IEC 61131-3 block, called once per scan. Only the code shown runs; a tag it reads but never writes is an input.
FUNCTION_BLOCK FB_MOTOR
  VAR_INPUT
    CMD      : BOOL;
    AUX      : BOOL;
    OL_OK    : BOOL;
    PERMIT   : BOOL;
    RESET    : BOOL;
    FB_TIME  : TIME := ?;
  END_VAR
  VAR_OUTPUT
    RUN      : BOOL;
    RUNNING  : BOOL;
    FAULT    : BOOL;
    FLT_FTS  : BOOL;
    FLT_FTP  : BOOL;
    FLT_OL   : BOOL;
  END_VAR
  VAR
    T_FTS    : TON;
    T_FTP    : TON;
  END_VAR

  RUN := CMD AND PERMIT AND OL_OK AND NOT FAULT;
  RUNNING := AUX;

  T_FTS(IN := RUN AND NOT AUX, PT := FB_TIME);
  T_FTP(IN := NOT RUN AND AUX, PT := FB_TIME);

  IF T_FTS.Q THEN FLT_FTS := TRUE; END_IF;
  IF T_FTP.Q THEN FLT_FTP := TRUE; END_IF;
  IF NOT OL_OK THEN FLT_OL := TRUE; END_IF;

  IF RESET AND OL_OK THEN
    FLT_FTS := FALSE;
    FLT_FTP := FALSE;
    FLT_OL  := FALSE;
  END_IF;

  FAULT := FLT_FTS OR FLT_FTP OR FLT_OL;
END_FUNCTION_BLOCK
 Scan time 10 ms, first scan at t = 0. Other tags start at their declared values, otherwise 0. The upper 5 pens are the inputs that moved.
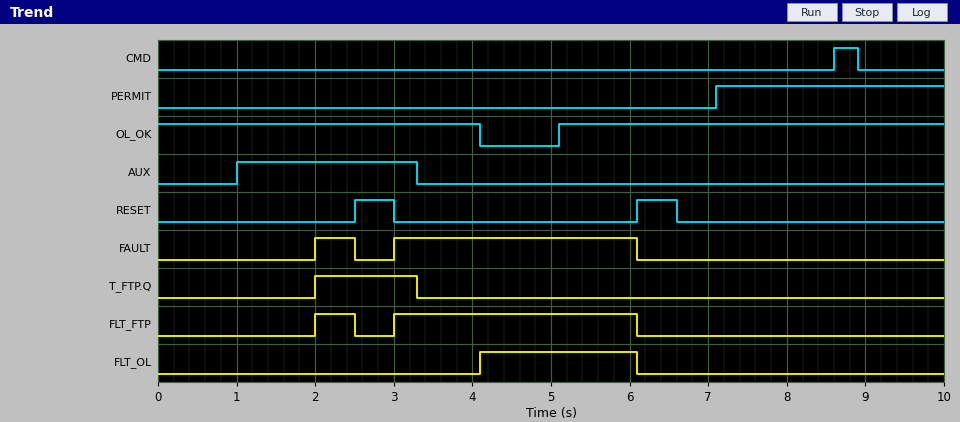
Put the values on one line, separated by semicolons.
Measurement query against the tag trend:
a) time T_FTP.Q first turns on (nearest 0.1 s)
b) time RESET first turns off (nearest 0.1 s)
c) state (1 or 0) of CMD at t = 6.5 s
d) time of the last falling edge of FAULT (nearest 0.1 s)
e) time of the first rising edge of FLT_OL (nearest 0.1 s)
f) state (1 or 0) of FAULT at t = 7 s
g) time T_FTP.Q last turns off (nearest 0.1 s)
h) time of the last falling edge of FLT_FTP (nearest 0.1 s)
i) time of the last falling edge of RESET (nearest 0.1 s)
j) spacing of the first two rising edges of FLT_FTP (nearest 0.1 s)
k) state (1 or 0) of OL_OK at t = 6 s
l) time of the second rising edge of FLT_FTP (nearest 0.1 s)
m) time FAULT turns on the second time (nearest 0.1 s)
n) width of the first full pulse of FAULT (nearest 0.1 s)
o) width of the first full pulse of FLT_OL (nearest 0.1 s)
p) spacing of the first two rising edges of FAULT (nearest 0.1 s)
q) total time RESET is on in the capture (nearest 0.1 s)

2.0 s; 3.0 s; 0; 6.1 s; 4.1 s; 0; 3.3 s; 6.1 s; 6.6 s; 1.0 s; 1; 3.0 s; 3.0 s; 0.5 s; 2.0 s; 1.0 s; 1.0 s
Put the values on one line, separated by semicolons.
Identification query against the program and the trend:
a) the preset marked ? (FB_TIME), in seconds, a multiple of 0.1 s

1.0 s
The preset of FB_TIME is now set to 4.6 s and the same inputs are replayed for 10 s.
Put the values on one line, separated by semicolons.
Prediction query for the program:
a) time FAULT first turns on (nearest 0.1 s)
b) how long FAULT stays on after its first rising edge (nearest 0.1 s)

4.1 s; 2.0 s
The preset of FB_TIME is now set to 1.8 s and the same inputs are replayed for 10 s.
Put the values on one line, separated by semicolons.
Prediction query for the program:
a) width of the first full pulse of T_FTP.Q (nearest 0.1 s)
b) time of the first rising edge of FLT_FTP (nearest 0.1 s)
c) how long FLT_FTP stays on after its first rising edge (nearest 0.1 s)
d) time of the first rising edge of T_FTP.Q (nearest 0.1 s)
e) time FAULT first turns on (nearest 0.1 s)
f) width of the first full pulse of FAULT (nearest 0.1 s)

0.5 s; 3.0 s; 3.1 s; 2.8 s; 3.0 s; 3.1 s
